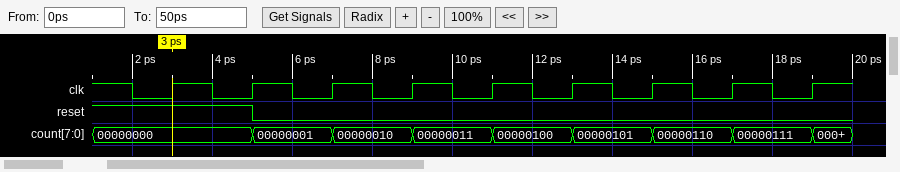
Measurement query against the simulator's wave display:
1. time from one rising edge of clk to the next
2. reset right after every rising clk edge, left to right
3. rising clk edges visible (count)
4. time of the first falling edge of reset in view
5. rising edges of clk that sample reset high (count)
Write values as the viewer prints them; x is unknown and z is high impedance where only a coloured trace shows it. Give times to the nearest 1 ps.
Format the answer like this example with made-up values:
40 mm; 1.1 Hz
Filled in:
2 ps; 1 0 0 0 0 0 0 0 0; 9; 5 ps; 2
